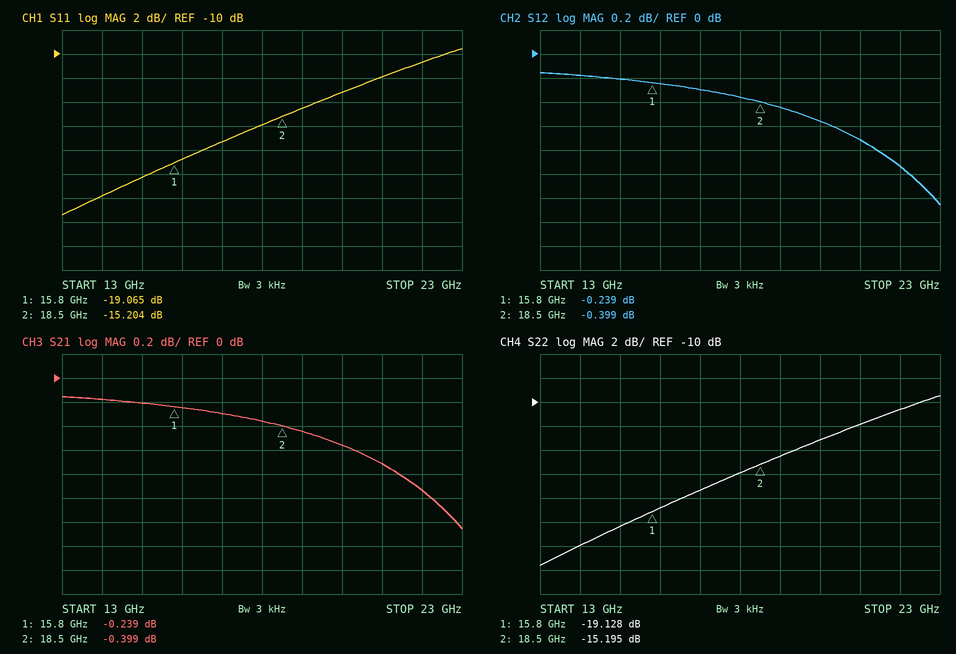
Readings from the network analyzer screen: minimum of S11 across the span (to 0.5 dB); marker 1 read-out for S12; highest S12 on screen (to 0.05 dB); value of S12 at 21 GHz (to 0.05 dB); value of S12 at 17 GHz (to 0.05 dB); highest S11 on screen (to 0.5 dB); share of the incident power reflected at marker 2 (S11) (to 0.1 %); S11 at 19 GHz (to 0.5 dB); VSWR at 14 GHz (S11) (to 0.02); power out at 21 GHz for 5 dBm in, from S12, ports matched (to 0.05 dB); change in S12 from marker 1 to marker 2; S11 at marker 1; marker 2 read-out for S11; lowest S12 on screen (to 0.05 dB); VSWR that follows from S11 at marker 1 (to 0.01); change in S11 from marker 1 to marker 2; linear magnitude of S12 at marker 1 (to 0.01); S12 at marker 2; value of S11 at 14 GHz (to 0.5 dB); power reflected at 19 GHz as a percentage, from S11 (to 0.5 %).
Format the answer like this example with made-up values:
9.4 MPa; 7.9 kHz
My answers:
-23.5 dB; -0.239 dB; -0.15 dB; -0.70 dB; -0.30 dB; -9.5 dB; 3.0 %; -14.5 dB; 1.18; 4.30 dBm; -0.160 dB; -19.065 dB; -15.204 dB; -1.25 dB; 1.25; 3.861 dB; 0.97; -0.399 dB; -22.0 dB; 3.5 %
